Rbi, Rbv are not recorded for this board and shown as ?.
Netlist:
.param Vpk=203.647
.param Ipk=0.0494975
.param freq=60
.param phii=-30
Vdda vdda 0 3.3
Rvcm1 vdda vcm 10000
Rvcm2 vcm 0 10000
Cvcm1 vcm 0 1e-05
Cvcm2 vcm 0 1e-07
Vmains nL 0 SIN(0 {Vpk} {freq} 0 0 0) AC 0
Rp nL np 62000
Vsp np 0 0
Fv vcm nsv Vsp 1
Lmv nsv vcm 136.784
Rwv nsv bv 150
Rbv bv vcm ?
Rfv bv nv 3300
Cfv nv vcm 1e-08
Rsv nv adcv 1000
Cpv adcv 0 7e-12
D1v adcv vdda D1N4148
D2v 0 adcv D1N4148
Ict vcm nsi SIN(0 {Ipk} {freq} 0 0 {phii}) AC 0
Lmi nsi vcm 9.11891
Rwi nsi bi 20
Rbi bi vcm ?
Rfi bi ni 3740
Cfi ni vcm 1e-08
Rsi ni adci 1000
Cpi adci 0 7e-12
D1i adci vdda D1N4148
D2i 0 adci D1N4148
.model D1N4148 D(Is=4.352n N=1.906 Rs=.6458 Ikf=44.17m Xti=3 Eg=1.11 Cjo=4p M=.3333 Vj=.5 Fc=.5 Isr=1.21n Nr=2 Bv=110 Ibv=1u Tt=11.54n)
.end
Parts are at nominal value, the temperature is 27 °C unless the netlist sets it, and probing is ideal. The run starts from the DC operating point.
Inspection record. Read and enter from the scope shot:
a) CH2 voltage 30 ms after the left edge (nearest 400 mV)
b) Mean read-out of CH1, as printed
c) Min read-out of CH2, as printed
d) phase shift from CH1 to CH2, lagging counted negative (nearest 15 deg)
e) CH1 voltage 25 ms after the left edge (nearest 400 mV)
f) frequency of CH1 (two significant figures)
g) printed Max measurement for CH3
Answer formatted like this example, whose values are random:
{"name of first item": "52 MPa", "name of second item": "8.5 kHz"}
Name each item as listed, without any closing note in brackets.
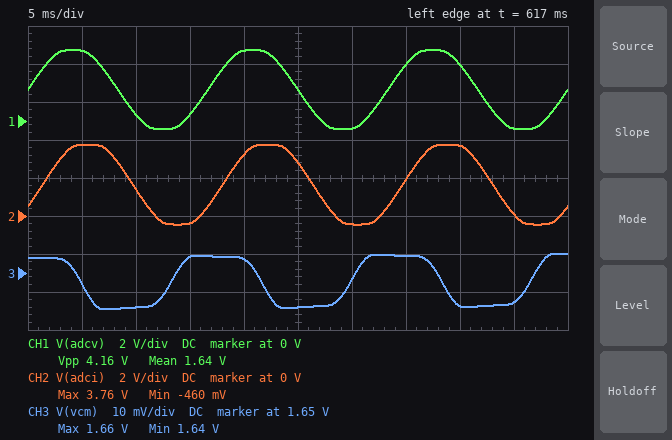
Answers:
{"CH2 voltage 30 ms after the left edge": "-400 mV", "Mean read-out of CH1, as printed": "1.64 V", "Min read-out of CH2, as printed": "-460 mV", "phase shift from CH1 to CH2, lagging counted negative": "-30 deg", "CH1 voltage 25 ms after the left edge": "1.6 V", "frequency of CH1": "60 Hz", "printed Max measurement for CH3": "1.66 V"}
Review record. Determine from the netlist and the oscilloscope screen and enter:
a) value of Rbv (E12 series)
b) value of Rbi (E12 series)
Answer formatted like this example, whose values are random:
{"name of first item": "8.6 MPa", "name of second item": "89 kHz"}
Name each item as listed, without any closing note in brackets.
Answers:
{"value of Rbv": "680 Ω", "value of Rbi": "47 Ω"}
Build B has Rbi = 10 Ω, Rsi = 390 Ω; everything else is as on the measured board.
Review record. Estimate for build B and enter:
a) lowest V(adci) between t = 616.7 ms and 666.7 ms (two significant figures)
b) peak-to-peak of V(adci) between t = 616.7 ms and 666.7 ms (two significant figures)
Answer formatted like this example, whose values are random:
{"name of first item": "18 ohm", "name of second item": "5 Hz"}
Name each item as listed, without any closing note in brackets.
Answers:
{"lowest V(adci) between t = 616.7 ms and 666.7 ms": "1.2 V", "peak-to-peak of V(adci) between t = 616.7 ms and 666.7 ms": "990 mV"}
